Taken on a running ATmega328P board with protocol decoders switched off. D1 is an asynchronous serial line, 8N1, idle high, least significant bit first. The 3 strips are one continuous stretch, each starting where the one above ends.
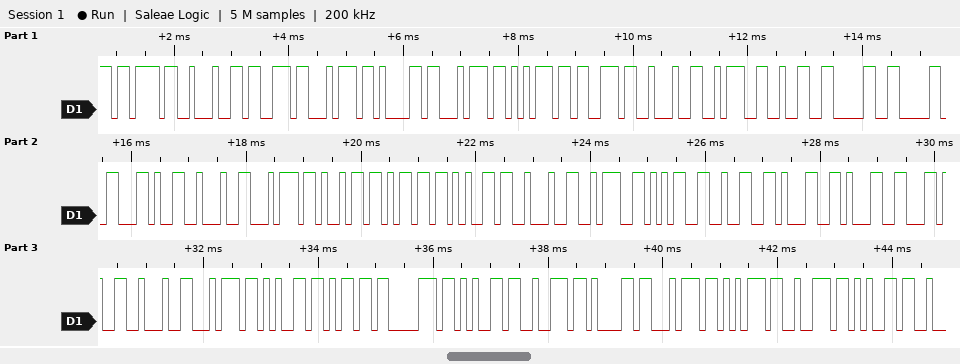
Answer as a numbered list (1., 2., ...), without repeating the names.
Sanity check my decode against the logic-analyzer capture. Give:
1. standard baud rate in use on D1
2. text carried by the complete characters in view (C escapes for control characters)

1. 9600 baud
2. "{\"status\":200,\"time\":5211,\"temperature"
